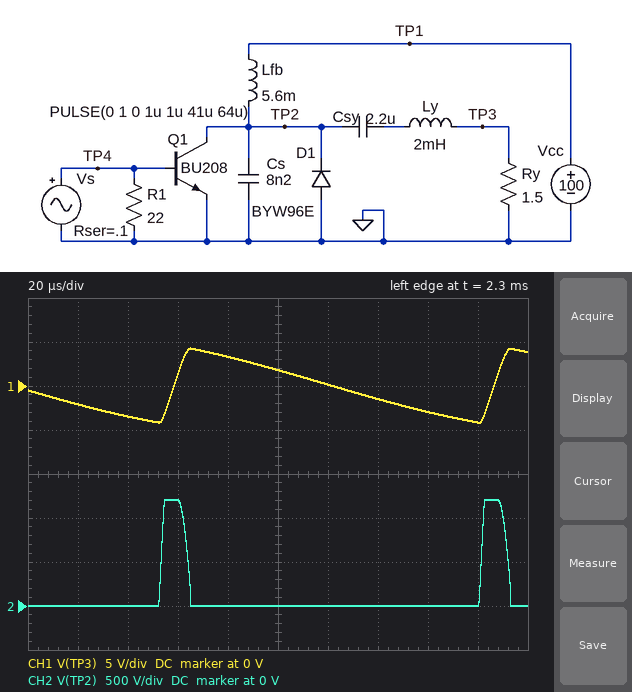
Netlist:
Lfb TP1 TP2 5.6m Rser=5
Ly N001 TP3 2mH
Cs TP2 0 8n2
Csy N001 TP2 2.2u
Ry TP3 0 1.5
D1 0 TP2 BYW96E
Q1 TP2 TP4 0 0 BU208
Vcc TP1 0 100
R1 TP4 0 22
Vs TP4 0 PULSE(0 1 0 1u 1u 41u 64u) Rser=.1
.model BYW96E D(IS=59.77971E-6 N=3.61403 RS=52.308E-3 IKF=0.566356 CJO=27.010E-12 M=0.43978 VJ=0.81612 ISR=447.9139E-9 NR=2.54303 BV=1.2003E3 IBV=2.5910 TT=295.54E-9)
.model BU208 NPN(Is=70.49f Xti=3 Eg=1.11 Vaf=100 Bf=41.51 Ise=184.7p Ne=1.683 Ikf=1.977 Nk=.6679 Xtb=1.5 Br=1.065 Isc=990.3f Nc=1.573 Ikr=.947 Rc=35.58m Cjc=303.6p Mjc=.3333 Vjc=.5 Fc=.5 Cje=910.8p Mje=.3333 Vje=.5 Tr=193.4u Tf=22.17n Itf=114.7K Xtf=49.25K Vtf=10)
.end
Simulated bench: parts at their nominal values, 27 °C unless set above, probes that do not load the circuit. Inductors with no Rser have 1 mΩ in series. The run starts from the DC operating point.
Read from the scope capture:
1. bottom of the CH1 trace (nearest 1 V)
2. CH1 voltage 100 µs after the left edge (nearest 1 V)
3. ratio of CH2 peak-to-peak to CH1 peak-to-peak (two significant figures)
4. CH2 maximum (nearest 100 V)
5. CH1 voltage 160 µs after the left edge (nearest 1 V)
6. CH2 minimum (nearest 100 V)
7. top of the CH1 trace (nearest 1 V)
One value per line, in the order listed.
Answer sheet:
-4 V
2 V
140
1.2 kV
-3 V
0 V
4 V
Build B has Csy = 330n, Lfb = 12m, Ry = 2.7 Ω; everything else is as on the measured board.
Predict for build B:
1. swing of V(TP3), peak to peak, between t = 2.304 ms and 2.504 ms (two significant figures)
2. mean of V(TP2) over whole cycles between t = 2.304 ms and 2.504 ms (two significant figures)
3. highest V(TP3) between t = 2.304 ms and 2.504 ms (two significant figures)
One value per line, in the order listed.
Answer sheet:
26 V
92 V
13 V
